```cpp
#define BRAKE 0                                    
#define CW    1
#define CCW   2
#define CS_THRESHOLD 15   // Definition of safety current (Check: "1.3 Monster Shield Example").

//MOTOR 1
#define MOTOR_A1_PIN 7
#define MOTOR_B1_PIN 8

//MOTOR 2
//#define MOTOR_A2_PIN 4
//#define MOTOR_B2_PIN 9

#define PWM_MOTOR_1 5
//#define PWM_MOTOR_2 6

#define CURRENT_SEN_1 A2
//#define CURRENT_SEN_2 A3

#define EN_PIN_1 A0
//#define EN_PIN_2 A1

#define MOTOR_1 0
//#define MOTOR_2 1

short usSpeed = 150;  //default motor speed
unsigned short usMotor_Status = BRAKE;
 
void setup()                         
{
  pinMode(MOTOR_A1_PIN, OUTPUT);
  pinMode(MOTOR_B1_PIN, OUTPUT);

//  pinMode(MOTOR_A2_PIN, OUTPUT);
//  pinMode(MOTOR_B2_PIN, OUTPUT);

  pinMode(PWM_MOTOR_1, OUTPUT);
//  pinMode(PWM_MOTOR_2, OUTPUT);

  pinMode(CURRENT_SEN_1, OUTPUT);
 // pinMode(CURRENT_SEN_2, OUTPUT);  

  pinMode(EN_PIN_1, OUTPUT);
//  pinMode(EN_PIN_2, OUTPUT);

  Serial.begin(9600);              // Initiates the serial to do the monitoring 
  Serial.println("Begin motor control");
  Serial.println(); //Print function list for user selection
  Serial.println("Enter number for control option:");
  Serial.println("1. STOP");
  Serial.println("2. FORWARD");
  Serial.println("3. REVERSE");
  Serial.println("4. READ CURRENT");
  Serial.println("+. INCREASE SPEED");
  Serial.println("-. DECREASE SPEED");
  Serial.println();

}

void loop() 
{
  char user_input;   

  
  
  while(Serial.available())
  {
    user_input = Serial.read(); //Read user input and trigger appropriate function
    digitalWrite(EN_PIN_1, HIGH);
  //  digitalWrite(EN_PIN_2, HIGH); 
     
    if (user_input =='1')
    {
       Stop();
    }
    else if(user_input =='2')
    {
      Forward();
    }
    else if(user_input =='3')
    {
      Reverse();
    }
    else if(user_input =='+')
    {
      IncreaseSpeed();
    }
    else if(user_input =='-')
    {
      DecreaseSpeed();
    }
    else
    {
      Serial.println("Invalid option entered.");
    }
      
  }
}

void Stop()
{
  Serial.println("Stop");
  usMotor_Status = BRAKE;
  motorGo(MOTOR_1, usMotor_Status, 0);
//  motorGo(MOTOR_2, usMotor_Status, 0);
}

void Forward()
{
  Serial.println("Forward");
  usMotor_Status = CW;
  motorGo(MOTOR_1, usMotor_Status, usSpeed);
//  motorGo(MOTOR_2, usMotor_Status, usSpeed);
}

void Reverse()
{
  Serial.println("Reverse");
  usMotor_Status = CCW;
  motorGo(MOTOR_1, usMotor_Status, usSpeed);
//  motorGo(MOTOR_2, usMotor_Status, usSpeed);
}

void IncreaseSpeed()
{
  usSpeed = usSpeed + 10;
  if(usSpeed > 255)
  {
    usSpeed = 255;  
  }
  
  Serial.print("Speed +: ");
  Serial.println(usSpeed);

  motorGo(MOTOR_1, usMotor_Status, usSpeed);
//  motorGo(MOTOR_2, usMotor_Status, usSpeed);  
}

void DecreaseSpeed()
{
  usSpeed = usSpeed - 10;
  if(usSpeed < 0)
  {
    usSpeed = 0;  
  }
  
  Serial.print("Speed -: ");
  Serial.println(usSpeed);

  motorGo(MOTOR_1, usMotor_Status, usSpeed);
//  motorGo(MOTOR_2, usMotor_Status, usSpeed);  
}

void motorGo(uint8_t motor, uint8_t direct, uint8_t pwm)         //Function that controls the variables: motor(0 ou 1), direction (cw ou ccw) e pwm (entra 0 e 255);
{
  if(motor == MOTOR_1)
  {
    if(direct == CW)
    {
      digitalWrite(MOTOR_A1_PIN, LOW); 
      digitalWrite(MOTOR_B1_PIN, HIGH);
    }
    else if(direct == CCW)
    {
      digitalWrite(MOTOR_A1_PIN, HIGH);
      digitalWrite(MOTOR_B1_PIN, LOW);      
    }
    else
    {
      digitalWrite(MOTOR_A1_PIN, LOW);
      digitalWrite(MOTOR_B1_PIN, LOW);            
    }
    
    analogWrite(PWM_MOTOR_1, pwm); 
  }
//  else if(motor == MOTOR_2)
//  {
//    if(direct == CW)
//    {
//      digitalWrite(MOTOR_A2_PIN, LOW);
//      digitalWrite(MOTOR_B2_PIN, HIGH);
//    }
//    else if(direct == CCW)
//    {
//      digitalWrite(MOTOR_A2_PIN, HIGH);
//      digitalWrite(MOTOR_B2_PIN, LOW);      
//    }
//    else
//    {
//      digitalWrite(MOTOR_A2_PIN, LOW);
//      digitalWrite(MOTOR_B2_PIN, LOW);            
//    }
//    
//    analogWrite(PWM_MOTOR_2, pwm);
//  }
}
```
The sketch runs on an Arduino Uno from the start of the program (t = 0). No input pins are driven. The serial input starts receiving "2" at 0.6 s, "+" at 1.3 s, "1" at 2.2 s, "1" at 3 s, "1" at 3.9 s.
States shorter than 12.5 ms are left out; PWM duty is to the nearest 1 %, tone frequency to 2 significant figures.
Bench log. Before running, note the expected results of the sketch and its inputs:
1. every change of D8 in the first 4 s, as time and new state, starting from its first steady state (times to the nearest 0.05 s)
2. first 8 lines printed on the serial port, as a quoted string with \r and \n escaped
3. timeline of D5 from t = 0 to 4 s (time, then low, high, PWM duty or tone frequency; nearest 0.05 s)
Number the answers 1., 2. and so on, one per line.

1. 0 s low; 0.6 s high; 2.2 s low
2. "Begin motor control\r\n\r\nEnter number for control option:\r\n1. STOP\r\n2. FORWARD\r\n3. REVERSE\r\n4. READ CURRENT\r\n+. INCREASE SPEED\r\n"
3. 0 s low; 0.6 s PWM 59 %; 1.3 s PWM 63 %; 2.2 s low
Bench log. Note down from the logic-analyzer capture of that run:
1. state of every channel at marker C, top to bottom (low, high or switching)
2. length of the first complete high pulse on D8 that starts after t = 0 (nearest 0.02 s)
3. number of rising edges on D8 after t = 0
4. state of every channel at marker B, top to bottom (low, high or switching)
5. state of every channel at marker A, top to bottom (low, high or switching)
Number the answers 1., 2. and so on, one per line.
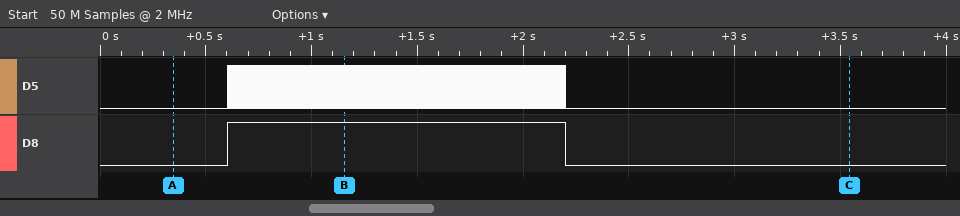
1. D5 low, D8 low
2. 1.60 s
3. 1
4. D5 switching, D8 high
5. D5 low, D8 low
